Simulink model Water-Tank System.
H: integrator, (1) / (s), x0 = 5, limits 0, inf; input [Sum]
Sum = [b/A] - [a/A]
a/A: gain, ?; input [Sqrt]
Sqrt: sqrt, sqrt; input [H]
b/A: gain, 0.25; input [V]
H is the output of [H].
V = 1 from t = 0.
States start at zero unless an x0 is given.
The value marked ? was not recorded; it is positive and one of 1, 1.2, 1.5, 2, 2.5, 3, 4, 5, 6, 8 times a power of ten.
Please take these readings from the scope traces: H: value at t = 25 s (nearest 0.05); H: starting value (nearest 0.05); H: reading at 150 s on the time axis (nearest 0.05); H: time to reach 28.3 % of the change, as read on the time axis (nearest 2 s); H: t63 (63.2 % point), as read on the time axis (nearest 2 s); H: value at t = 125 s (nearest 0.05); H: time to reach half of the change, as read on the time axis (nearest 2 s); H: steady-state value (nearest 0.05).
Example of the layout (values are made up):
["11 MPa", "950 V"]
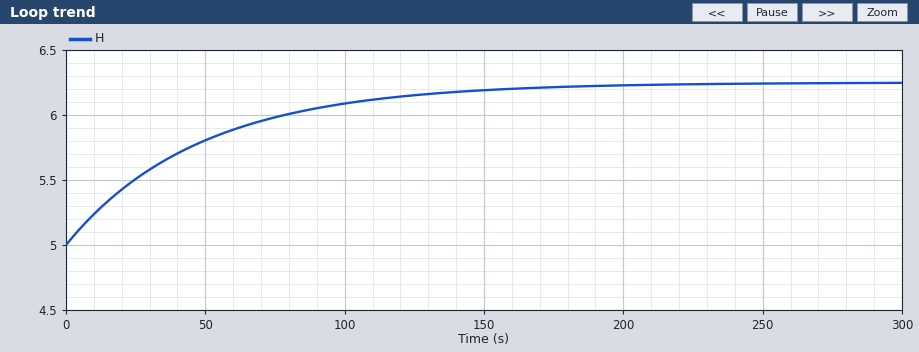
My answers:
["5.50", "5.00", "6.20", "16 s", "48 s", "6.15", "34 s", "6.25"]
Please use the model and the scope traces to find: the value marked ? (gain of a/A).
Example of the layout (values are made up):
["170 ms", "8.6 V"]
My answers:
["0.1"]
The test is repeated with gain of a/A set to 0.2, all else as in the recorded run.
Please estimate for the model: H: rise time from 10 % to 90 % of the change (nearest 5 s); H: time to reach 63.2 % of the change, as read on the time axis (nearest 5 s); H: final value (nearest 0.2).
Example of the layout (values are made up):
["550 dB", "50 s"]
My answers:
["30 s", "15 s", "1.6"]
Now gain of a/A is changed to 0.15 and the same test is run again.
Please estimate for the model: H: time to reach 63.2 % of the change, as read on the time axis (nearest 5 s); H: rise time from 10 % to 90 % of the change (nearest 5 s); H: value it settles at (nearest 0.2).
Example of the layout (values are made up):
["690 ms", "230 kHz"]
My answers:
["25 s", "50 s", "2.8"]
